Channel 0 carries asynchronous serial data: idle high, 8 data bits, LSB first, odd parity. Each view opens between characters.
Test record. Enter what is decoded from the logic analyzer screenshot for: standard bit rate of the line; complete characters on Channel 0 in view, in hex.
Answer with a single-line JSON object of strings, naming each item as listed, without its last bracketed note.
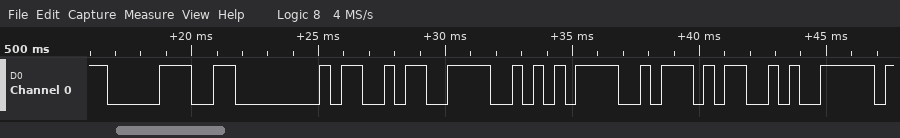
{"standard bit rate of the line": "2400 baud", "complete characters on Channel 0 in view, in hex": "70, 80, 9A, AA, BA, CA"}
